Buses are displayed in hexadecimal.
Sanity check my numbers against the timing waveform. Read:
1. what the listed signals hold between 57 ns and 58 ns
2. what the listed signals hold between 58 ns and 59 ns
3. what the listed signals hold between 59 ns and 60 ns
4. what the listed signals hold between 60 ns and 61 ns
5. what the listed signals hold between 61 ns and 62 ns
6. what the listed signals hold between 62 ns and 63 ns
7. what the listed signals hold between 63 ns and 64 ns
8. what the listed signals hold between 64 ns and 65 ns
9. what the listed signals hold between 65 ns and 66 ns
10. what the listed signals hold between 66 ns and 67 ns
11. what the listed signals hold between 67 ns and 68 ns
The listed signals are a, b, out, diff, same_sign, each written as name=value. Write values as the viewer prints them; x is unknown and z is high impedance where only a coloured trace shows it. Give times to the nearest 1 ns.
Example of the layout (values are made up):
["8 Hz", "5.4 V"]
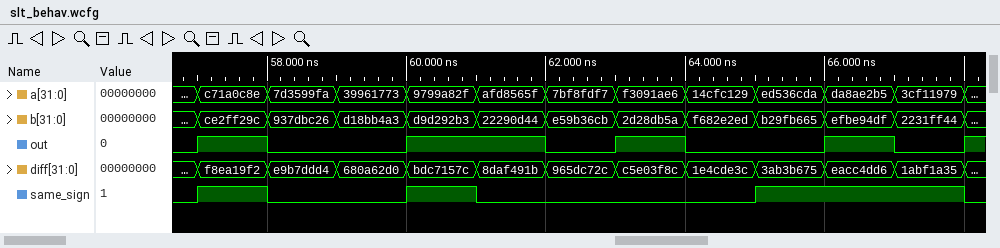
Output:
["a=c71a0c8e, b=ce2ff29c, out=1, diff=f8ea19f2, same_sign=1", "a=7d3599fa, b=937dbc26, out=0, diff=e9b7ddd4, same_sign=0", "a=39961773, b=d18bb4a3, out=0, diff=680a62d0, same_sign=0", "a=9799a82f, b=d9d292b3, out=1, diff=bdc7157c, same_sign=1", "a=afd8565f, b=22290d44, out=1, diff=8daf491b, same_sign=0", "a=7bf8fdf7, b=e59b36cb, out=0, diff=965dc72c, same_sign=0", "a=f3091ae6, b=2d28db5a, out=1, diff=c5e03f8c, same_sign=0", "a=14cfc129, b=f682e2ed, out=0, diff=1e4cde3c, same_sign=0", "a=ed536cda, b=b29fb665, out=0, diff=3ab3b675, same_sign=1", "a=da8ae2b5, b=efbe94df, out=1, diff=eacc4dd6, same_sign=1", "a=3cf11979, b=2231ff44, out=0, diff=1abf1a35, same_sign=1"]
